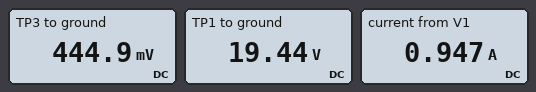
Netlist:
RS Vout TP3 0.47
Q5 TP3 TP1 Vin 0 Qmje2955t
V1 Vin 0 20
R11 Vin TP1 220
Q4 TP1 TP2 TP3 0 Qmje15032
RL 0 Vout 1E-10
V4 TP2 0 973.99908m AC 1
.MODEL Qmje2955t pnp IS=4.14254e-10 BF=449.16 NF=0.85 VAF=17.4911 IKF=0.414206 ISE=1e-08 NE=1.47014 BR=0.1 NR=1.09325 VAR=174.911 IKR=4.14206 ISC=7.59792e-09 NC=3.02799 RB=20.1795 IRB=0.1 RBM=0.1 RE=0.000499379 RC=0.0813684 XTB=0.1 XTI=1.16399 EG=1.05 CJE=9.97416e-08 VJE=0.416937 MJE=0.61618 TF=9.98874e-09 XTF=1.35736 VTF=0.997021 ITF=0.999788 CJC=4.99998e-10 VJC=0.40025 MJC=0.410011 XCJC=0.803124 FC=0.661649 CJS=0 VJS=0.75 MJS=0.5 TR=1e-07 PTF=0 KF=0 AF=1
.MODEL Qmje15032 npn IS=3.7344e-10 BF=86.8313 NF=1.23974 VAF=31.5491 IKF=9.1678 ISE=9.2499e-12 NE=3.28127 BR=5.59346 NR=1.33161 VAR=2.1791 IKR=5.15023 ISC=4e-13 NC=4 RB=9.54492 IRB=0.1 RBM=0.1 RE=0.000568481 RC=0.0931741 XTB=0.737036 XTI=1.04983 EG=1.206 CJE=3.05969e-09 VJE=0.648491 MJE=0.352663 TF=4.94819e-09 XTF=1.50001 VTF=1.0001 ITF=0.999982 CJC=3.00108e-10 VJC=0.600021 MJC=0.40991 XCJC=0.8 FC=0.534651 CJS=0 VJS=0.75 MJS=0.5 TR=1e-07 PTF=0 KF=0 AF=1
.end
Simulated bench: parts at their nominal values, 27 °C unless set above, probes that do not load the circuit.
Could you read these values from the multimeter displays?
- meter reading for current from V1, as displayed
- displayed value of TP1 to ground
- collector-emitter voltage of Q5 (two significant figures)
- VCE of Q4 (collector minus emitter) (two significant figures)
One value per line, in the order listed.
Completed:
0.947 A
19.44 V
-20 V
19 V
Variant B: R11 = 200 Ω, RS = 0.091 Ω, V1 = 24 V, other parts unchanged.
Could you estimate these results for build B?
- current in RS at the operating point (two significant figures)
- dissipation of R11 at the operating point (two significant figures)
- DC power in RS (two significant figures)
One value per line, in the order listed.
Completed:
4.3 A
4.8 mW
1.7 W
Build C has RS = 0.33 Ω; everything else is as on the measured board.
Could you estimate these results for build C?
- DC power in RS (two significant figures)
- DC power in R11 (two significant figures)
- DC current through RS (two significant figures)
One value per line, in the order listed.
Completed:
570 mW
1.7 mW
1.3 A
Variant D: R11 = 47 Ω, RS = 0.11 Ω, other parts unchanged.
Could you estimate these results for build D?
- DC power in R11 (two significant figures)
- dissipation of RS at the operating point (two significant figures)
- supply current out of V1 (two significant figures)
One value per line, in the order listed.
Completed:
18 mW
1.3 W
3.5 A
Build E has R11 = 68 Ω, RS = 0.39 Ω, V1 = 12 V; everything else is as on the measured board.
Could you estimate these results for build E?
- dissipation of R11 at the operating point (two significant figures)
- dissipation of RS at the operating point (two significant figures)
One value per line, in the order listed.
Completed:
5.5 mW
430 mW
